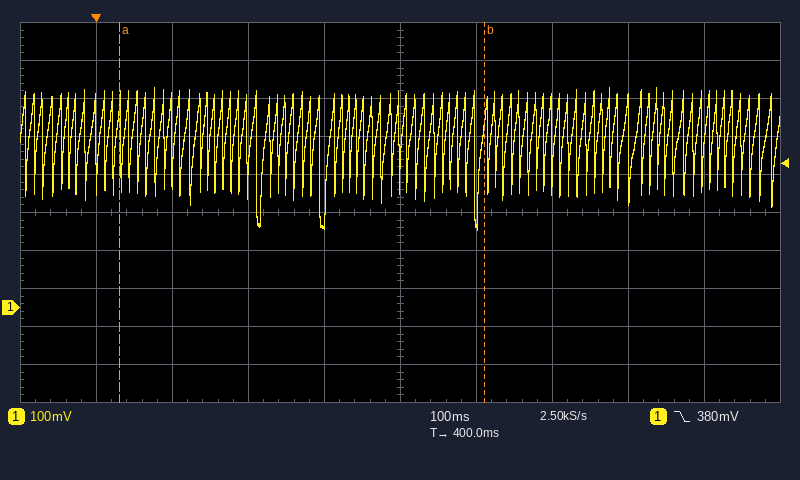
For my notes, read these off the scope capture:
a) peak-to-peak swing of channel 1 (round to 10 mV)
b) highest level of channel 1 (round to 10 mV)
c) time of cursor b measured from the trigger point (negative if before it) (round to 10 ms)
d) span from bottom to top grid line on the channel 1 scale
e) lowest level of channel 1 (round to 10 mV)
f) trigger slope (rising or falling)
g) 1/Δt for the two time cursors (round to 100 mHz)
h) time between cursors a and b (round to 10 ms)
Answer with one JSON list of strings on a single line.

["370 mV", "580 mV", "+510 ms", "1 V", "210 mV", "falling", "2.1 Hz", "480 ms"]
